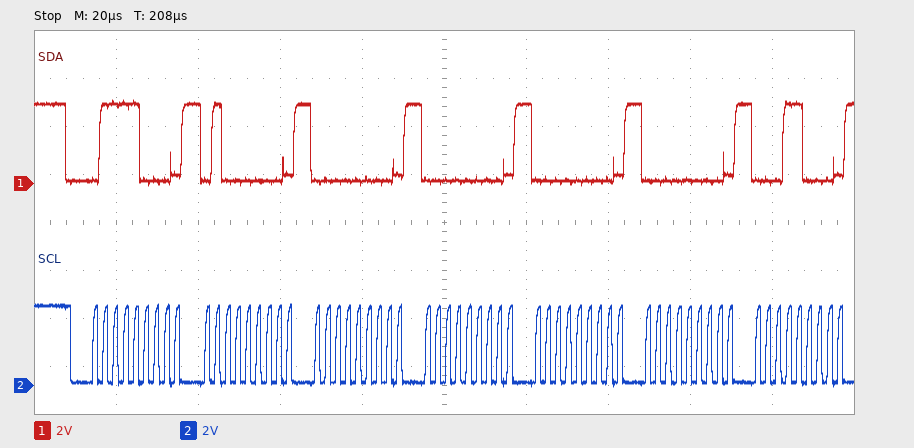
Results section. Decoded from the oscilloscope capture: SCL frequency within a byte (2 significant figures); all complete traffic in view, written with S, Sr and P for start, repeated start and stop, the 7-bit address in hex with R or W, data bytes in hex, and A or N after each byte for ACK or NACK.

400 kHz
S 3CW A 40 A 00 A 00 A 00 A 00 A 18 A
